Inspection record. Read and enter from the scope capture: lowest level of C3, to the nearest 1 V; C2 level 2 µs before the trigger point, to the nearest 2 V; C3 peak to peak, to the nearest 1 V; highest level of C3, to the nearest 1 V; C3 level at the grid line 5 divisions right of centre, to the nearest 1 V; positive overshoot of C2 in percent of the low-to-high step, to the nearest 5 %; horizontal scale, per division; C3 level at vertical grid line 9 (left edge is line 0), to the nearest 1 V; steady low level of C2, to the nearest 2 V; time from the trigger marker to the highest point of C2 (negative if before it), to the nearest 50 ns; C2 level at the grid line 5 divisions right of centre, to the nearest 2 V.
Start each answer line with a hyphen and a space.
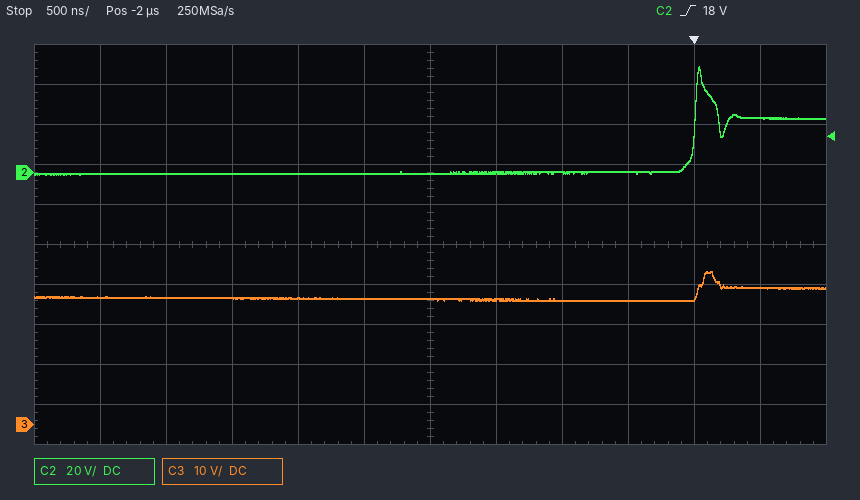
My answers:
- 31 V
- 0 V
- 7 V
- 38 V
- 34 V
- 95 %
- 500 ns
- 31 V
- 0 V
- +50 ns
- 28 V
